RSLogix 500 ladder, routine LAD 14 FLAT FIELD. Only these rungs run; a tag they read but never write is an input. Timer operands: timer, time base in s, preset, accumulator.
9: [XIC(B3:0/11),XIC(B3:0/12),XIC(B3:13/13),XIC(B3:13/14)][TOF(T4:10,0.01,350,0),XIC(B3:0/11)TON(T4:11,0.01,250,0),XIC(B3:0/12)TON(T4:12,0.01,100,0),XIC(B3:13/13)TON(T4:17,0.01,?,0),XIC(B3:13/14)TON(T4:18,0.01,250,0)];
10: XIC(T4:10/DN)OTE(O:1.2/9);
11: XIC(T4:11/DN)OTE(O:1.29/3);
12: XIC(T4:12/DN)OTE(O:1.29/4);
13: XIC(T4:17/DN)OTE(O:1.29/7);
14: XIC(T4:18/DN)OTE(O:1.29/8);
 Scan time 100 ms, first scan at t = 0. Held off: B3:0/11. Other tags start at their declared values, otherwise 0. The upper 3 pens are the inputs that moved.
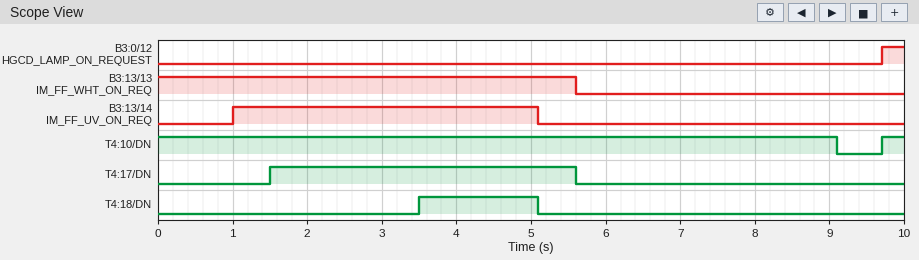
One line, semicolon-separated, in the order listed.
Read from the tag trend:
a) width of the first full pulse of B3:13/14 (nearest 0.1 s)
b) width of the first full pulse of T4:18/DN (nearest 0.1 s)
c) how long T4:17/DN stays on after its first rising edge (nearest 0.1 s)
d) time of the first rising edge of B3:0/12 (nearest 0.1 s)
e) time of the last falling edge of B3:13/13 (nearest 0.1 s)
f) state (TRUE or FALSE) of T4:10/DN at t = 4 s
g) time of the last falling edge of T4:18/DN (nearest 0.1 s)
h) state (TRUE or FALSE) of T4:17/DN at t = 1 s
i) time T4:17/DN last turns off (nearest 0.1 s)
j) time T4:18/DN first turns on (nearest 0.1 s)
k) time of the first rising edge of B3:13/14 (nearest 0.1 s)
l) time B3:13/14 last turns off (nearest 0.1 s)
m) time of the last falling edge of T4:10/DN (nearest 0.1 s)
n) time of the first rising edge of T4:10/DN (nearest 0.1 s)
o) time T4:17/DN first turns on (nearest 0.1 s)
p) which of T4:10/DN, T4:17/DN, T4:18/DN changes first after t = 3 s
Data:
4.1 s; 1.6 s; 4.1 s; 9.7 s; 5.6 s; TRUE; 5.1 s; FALSE; 5.6 s; 3.5 s; 1.0 s; 5.1 s; 9.1 s; 9.7 s; 1.5 s; T4:18/DN
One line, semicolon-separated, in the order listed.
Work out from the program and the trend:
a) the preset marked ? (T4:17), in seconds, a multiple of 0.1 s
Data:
1.5 s
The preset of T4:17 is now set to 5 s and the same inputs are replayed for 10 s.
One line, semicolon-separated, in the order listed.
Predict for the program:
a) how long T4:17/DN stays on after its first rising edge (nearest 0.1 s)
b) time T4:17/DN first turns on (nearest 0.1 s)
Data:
0.6 s; 5.0 s
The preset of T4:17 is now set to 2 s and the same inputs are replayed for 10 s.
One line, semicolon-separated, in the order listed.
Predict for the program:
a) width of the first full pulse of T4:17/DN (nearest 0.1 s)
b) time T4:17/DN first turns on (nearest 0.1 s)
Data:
3.6 s; 2.0 s
